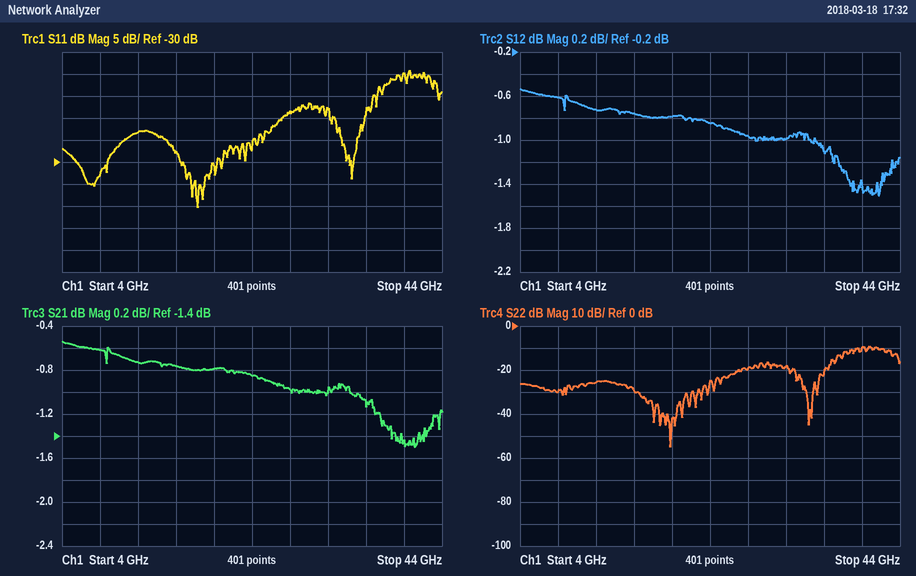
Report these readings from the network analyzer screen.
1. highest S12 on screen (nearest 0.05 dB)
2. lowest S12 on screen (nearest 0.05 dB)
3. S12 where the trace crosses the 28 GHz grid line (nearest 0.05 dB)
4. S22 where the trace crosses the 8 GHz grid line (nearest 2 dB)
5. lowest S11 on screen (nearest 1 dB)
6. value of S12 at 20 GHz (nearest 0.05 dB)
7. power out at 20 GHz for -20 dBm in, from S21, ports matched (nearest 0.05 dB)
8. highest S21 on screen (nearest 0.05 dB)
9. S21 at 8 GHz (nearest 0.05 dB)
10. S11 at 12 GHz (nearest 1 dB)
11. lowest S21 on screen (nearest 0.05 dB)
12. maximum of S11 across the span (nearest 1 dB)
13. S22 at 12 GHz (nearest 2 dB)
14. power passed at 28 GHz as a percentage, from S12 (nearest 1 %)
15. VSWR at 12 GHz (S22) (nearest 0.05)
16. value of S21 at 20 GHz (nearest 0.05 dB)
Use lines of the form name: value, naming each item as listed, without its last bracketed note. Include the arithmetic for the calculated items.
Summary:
highest S12 on screen: -0.55 dB
lowest S12 on screen: -1.50 dB
S12 where the trace crosses the 28 GHz grid line: -0.95 dB
S22 where the trace crosses the 8 GHz grid line: -30 dB
lowest S11 on screen: -40 dB
value of S12 at 20 GHz: -0.80 dB
power out at 20 GHz for -20 dBm in, from S21, ports matched: -20 dBm + (-0.80 dB) = -20.80 dBm
highest S21 on screen: -0.55 dB
S21 at 8 GHz: -0.60 dB
S11 at 12 GHz: -23 dB
lowest S21 on screen: -1.50 dB
maximum of S11 across the span: -9 dB
S22 at 12 GHz: -26 dB
power passed at 28 GHz as a percentage, from S12: 10^(-0.95/10) ≈ 80 %
VSWR at 12 GHz (S22): |Γ| = 10^(-26/20) = 0.0501; VSWR = (1 + 0.0501)/(1 − 0.0501) ≈ 1.11, so 1.10 to the nearest 0.05
value of S21 at 20 GHz: -0.80 dB
